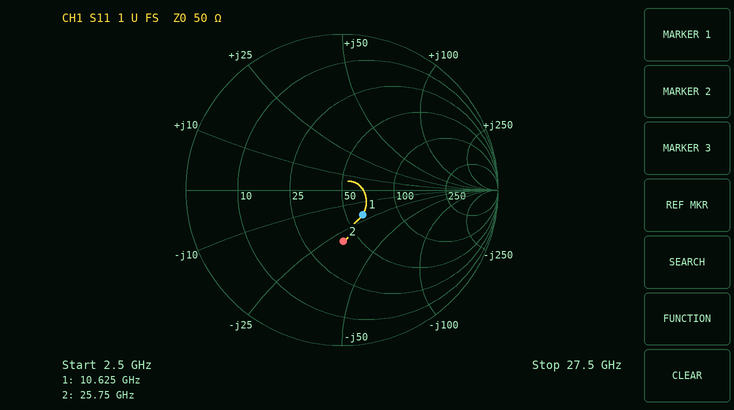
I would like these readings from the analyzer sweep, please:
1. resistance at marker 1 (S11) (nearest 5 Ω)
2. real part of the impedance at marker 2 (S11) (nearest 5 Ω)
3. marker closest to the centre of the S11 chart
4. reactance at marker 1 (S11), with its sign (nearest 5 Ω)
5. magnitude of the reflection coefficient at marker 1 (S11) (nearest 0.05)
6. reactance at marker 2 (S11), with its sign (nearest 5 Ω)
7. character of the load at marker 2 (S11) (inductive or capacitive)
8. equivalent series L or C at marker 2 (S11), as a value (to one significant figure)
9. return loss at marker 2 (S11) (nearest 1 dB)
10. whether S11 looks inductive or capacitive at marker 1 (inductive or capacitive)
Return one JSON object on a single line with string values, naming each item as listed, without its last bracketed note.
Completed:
{"resistance at marker 1 (S11)": "60 Ω", "real part of the impedance at marker 2 (S11)": "40 Ω", "marker closest to the centre of the S11 chart": "marker 1", "reactance at marker 1 (S11), with its sign": "-20 Ω", "magnitude of the reflection coefficient at marker 1 (S11)": "0.20", "reactance at marker 2 (S11), with its sign": "-30 Ω", "character of the load at marker 2 (S11)": "capacitive", "equivalent series L or C at marker 2 (S11), as a value": "200 fF", "return loss at marker 2 (S11)": "10 dB", "whether S11 looks inductive or capacitive at marker 1": "capacitive"}
